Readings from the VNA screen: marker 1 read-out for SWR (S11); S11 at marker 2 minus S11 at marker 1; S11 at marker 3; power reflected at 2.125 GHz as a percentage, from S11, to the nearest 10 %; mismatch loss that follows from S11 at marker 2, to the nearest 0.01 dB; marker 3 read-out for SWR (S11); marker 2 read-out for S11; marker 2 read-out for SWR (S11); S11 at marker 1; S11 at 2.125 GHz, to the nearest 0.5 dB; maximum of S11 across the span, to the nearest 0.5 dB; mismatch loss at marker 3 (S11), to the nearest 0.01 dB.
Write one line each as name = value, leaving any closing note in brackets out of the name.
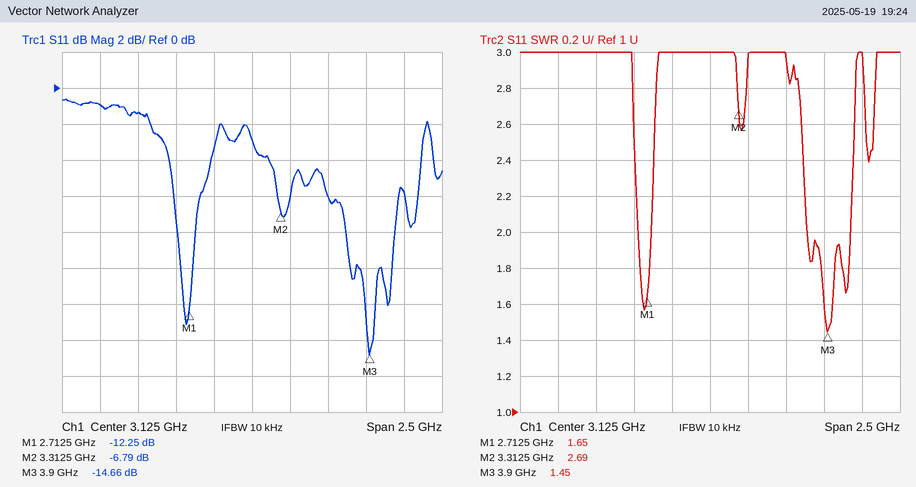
marker 1 read-out for SWR = 1.65
S11 at marker 2 minus S11 at marker 1 = 5.46 dB
S11 at marker 3 = -14.66 dB
power reflected at 2.125 GHz as a percentage, from S11, to the nearest 10 % = 80 %
mismatch loss that follows from S11 at marker 2, to the nearest 0.01 dB = 1.02 dB
marker 3 read-out for SWR = 1.45
marker 2 read-out for S11 = -6.79 dB
marker 2 read-out for SWR = 2.69
S11 at marker 1 = -12.25 dB
S11 at 2.125 GHz, to the nearest 0.5 dB = -1.0 dB
maximum of S11 across the span, to the nearest 0.5 dB = -0.5 dB
mismatch loss at marker 3 (S11), to the nearest 0.01 dB = 0.15 dB
